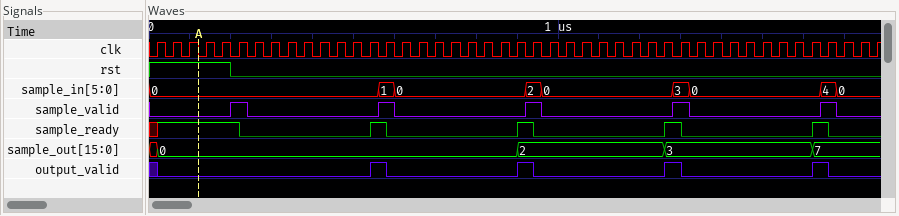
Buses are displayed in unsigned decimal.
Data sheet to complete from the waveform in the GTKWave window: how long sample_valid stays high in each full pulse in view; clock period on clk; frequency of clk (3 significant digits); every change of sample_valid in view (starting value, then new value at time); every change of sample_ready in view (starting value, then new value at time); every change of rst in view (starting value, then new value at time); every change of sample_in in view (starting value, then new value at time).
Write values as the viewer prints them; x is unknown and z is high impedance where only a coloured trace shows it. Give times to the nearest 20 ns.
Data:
40 ns, 40 ns, 40 ns, 40 ns, 40 ns
40 ns
25.0 MHz
0, 1 at 200 ns, 0 at 240 ns, 1 at 560 ns, 0 at 600 ns, 1 at 920 ns, 0 at 960 ns, 1 at 1280 ns, 0 at 1320 ns, 1 at 1640 ns, 0 at 1680 ns
x, 1 at 20 ns, 0 at 220 ns, 1 at 540 ns, 0 at 580 ns, 1 at 900 ns, 0 at 940 ns, 1 at 1260 ns, 0 at 1300 ns, 1 at 1620 ns, 0 at 1660 ns
1, 0 at 200 ns
0, 1 at 560 ns, 0 at 600 ns, 2 at 920 ns, 0 at 960 ns, 3 at 1280 ns, 0 at 1320 ns, 4 at 1640 ns, 0 at 1680 ns
